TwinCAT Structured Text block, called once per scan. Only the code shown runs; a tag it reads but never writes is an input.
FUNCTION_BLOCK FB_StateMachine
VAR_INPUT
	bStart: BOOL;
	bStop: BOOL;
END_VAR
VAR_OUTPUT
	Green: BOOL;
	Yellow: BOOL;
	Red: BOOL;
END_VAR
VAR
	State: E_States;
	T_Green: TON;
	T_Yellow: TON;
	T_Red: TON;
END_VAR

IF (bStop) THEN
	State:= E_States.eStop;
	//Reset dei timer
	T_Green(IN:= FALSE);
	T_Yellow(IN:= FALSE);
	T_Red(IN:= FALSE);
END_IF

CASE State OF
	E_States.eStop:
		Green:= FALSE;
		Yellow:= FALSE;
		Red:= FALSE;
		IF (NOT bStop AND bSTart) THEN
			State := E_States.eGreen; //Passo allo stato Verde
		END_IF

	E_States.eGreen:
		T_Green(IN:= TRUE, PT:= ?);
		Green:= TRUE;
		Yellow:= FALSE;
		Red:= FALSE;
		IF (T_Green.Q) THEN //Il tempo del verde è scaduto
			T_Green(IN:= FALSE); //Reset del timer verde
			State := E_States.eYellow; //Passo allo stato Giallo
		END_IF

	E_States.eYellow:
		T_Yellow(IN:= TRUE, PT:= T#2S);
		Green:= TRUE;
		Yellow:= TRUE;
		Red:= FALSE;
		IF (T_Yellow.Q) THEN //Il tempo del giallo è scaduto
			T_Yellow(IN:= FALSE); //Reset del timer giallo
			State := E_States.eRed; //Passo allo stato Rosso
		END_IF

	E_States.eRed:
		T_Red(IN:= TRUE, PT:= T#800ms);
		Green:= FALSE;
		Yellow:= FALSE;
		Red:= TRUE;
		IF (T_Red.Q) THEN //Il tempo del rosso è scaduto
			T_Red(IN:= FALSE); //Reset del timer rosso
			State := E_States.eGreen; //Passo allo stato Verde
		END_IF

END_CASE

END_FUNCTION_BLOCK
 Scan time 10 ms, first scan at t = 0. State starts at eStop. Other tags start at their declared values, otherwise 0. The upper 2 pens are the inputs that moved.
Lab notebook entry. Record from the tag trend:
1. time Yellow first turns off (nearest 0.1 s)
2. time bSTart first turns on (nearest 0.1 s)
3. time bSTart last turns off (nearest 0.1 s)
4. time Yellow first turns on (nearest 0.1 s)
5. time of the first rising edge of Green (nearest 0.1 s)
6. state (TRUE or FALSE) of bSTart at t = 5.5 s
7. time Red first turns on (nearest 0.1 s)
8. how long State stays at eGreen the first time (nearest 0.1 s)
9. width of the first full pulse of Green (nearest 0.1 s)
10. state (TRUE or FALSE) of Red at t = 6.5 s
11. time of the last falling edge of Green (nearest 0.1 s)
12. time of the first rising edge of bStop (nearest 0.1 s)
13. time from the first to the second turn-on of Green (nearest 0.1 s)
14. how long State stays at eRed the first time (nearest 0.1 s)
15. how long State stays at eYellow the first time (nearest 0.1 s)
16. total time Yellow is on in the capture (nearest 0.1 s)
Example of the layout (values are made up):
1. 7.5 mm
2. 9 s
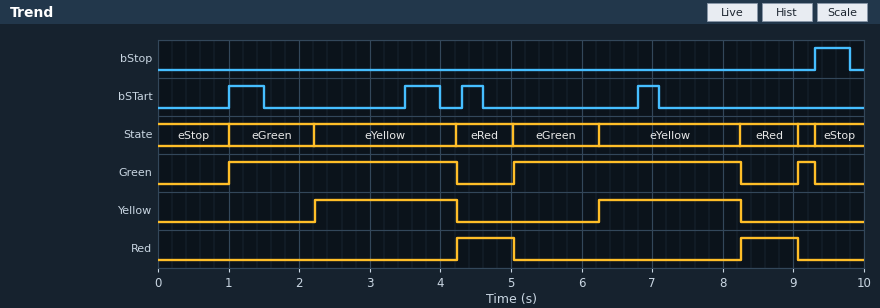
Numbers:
1. 4.2 s
2. 1.0 s
3. 7.1 s
4. 2.2 s
5. 1.0 s
6. FALSE
7. 4.2 s
8. 1.2 s
9. 3.2 s
10. FALSE
11. 9.3 s
12. 9.3 s
13. 4.0 s
14. 0.8 s
15. 2.0 s
16. 4.0 s
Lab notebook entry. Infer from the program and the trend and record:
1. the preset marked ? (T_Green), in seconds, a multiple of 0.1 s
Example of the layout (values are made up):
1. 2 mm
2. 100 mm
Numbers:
1. 1.2 s
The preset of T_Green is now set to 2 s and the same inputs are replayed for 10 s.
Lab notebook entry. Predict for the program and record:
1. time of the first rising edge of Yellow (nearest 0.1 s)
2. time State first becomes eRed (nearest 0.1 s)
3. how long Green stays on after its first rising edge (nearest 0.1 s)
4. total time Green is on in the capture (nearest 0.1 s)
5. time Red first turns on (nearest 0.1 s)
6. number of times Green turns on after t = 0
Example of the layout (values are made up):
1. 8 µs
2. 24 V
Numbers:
1. 3.0 s
2. 5.0 s
3. 4.0 s
4. 7.5 s
5. 5.0 s
6. 2
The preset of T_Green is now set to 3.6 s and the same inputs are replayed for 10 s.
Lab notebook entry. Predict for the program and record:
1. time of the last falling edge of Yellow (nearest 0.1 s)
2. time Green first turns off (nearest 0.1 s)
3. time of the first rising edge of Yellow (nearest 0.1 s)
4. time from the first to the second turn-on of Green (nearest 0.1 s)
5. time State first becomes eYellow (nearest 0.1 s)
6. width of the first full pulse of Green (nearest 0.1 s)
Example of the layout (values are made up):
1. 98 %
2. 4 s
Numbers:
1. 6.6 s
2. 6.6 s
3. 4.6 s
4. 6.4 s
5. 4.6 s
6. 5.6 s
